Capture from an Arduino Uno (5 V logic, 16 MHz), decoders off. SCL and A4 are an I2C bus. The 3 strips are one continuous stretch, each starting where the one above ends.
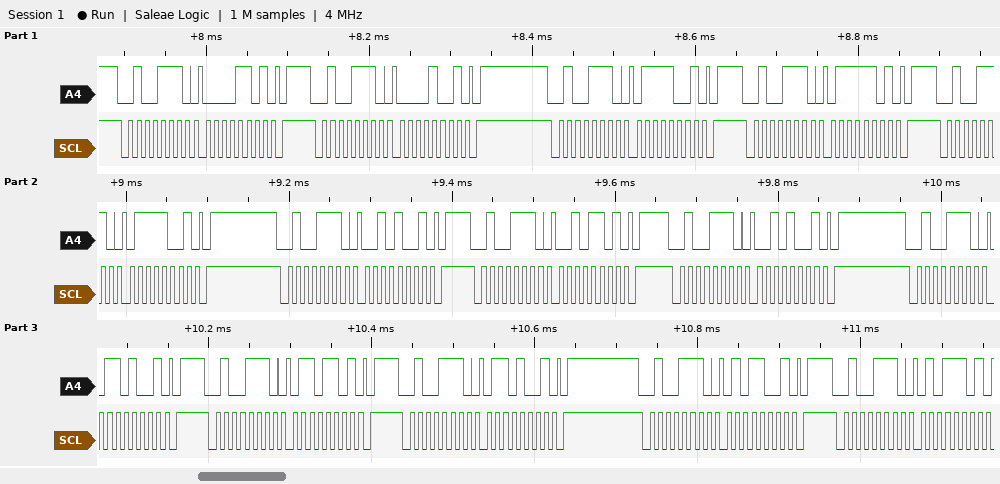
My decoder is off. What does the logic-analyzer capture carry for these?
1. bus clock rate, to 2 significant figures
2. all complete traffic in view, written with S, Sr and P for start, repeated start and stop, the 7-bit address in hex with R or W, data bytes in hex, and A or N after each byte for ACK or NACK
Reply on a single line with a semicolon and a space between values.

100 kHz; S 27W A 0D A P S 27W A 09 A P S 27W A 79 A P S 27W A 7D A P S 27W A 79 A P S 27W A 29 A P S 27W A 2D A P S 27W A 29 A P S 27W A 69 A P S 27W A 6D A P S 27W A 69 A P S 27W A 59 A P S 27W A 5D A
